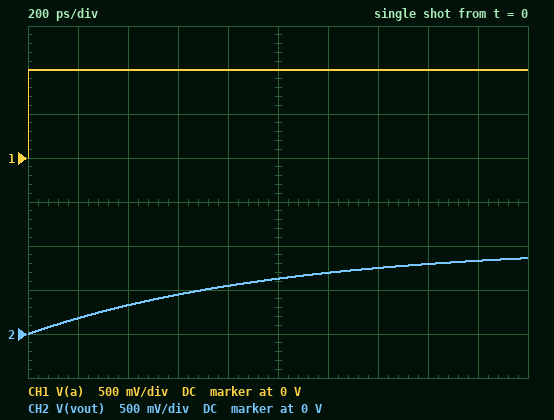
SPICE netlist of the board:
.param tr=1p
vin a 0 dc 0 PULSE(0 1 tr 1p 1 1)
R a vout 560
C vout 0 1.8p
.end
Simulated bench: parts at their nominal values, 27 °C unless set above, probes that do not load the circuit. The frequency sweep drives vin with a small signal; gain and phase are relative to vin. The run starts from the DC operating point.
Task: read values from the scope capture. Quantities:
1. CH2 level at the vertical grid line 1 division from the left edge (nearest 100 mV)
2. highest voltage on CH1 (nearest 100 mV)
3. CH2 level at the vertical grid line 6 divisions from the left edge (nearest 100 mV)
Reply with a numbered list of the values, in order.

1. 200 mV
2. 1.0 V
3. 700 mV
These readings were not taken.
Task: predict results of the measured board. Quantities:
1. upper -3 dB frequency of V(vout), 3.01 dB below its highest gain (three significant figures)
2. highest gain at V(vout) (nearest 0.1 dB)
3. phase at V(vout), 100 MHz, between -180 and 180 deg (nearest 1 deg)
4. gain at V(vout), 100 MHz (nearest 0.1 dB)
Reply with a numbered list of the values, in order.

1. 158 MHz
2. 0 dB
3. -32 deg
4. -1.5 dB
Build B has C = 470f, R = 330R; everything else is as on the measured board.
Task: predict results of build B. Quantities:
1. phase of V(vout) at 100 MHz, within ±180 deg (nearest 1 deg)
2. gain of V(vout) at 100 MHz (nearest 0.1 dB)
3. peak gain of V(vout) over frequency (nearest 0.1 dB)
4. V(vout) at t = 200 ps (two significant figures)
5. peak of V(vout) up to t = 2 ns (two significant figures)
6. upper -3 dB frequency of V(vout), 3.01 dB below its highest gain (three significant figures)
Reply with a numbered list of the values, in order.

1. -6 deg
2. 0 dB
3. 0 dB
4. 720 mV
5. 1.0 V
6. 1.03 GHz
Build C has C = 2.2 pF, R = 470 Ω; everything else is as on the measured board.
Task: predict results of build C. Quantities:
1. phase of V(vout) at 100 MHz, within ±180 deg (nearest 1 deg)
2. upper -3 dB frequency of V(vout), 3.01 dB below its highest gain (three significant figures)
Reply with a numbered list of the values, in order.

1. -33 deg
2. 154 MHz
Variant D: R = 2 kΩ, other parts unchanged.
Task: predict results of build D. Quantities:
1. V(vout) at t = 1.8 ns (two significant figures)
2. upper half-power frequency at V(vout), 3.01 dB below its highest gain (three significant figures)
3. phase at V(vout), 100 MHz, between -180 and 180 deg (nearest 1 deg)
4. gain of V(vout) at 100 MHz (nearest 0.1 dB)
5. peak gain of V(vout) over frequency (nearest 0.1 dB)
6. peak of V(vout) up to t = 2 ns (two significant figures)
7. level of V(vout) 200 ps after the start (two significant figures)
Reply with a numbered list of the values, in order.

1. 390 mV
2. 44.2 MHz
3. -66 deg
4. -7.9 dB
5. 0 dB
6. 430 mV
7. 54 mV
